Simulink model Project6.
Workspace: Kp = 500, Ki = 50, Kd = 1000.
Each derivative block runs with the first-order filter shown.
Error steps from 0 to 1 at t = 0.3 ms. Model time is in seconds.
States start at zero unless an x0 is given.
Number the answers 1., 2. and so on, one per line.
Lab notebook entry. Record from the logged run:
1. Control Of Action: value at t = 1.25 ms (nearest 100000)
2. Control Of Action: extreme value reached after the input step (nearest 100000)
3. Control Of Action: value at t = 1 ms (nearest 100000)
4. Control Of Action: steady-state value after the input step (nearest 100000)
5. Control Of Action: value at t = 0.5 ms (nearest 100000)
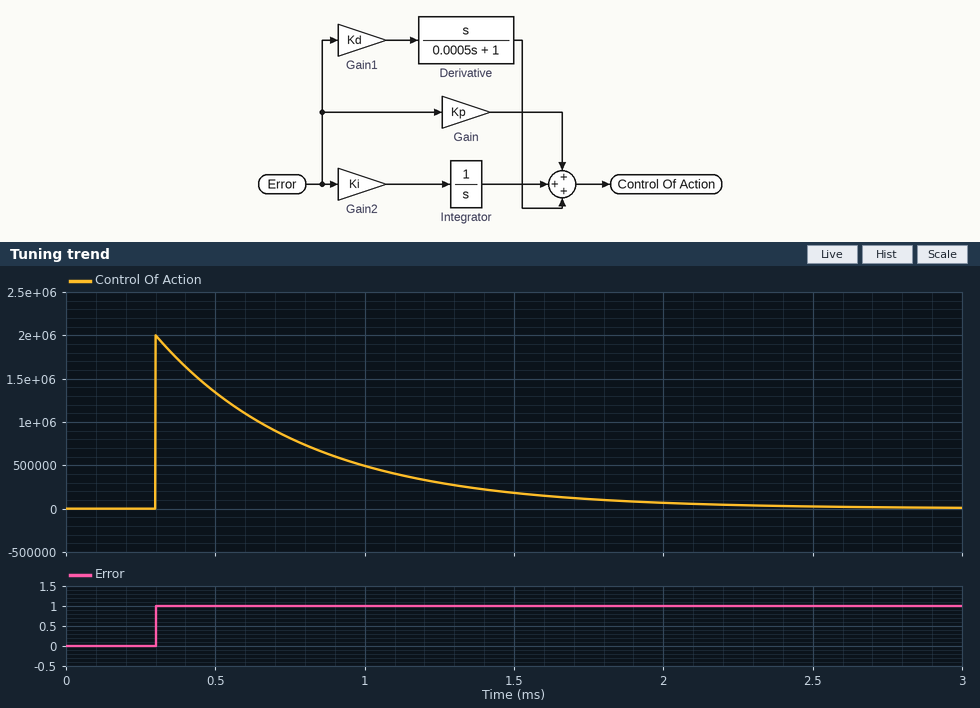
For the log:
1. 300000
2. 2000000
3. 500000
4. 0
5. 1300000
